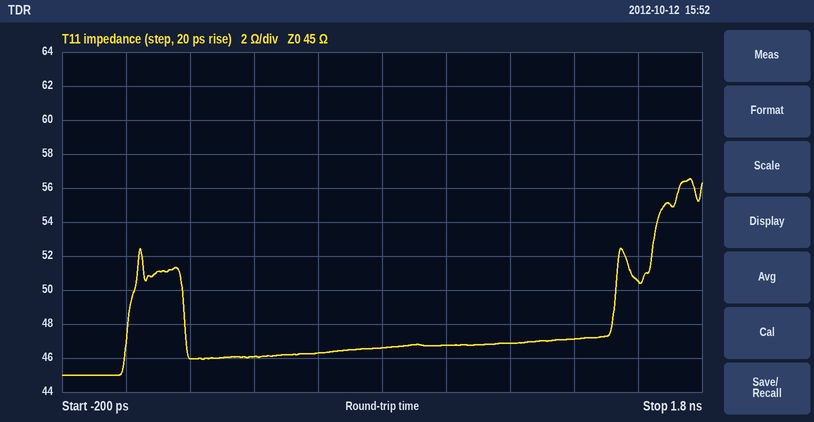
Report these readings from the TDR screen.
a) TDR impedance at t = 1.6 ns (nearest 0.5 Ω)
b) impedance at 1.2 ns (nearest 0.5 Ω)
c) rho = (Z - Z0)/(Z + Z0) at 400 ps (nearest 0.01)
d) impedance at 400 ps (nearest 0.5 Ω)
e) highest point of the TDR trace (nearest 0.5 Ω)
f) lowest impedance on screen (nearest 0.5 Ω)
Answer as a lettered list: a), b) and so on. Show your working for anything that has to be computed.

a) 50.5 Ω
b) 47.0 Ω
c) (46 − 45)/(46 + 45) ≈ +0.01
d) 46.0 Ω
e) 56.5 Ω
f) 45.0 Ω
